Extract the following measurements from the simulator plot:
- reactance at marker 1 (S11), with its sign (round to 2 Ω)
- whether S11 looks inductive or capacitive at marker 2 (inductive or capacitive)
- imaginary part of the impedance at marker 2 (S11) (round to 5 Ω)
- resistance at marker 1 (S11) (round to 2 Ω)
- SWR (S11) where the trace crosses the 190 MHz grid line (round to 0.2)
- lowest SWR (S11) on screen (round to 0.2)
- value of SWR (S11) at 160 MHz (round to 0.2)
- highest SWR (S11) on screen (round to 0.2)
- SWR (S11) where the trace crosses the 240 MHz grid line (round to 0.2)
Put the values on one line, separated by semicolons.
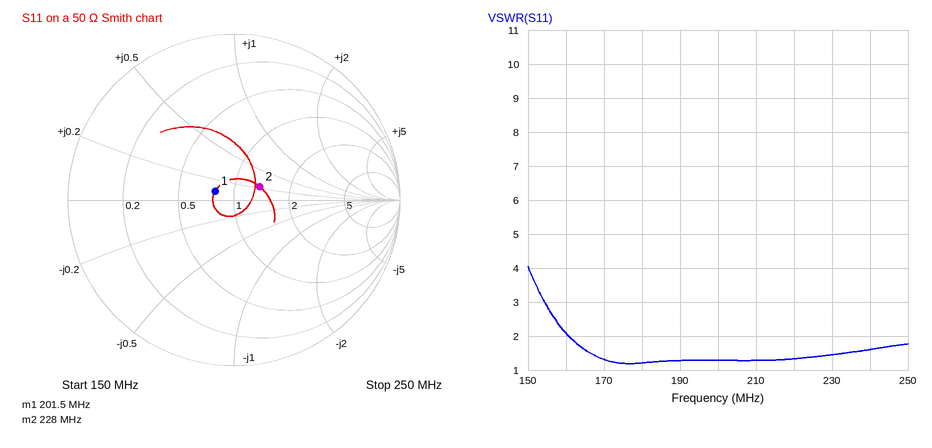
+4 Ω; inductive; +10 Ω; 40 Ω; 1.2; 1.2; 2.0; 4.0; 1.6
